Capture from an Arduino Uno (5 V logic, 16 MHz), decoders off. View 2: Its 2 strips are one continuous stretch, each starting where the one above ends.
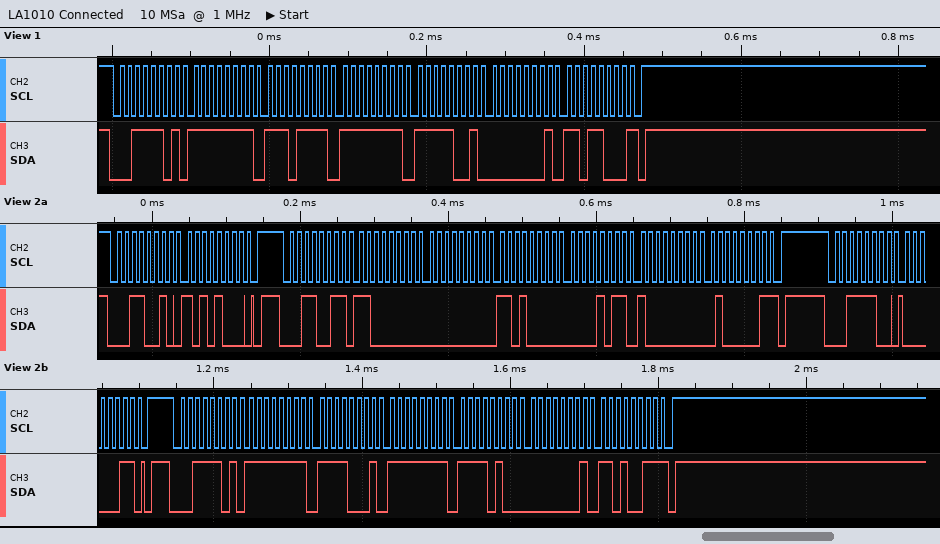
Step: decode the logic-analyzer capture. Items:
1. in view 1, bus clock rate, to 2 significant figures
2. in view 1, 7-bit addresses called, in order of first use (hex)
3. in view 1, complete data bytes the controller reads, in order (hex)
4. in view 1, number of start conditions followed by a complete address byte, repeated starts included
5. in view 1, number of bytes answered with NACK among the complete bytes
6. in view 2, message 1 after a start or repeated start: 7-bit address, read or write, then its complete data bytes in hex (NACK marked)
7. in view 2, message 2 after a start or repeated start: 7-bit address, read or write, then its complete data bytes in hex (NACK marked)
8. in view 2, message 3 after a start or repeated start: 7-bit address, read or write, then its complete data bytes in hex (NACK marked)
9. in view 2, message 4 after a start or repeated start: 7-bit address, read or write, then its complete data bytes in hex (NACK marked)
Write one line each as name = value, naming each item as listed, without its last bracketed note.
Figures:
in view 1, bus clock rate, to 2 significant figures = 100 kHz
in view 1, 7-bit addresses called, in order of first use = 0x1E
in view 1, complete data bytes the controller reads, in order = FF EF FF F9 01 D8
in view 1, number of start conditions followed by a complete address byte, repeated starts included = 1
in view 1, number of bytes answered with NACK among the complete bytes = 1
in view 2, message 1 after a start or repeated start: 7-bit address, read or write, then its complete data bytes in hex = 0x19 write: A8
in view 2, message 2 after a start or repeated start: 7-bit address, read or write, then its complete data bytes in hex = 0x19 read: C0 00 D0 0B 80 41 NACK
in view 2, message 3 after a start or repeated start: 7-bit address, read or write, then its complete data bytes in hex = 0x1E write: 03
in view 2, message 4 after a start or repeated start: 7-bit address, read or write, then its complete data bytes in hex = 0x1E read: FF F1 FF F4 01 D3 NACK
